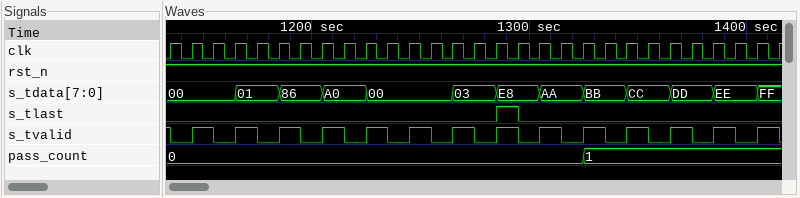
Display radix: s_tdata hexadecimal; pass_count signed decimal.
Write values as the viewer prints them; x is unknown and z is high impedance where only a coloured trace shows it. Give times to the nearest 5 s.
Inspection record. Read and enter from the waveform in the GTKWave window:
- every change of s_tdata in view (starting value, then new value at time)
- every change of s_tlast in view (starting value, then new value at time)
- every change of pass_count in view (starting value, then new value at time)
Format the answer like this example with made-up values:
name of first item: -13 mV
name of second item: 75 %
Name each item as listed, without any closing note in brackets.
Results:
every change of s_tdata in view: 00, 01 at 1165 s, 86 at 1185 s, A0 at 1205 s, 00 at 1225 s, 03 at 1265 s, E8 at 1285 s, AA at 1305 s, BB at 1325 s, CC at 1345 s, DD at 1365 s, EE at 1385 s, FF at 1405 s
every change of s_tlast in view: 0, 1 at 1285 s, 0 at 1295 s
every change of pass_count in view: 0, 1 at 1325 s
